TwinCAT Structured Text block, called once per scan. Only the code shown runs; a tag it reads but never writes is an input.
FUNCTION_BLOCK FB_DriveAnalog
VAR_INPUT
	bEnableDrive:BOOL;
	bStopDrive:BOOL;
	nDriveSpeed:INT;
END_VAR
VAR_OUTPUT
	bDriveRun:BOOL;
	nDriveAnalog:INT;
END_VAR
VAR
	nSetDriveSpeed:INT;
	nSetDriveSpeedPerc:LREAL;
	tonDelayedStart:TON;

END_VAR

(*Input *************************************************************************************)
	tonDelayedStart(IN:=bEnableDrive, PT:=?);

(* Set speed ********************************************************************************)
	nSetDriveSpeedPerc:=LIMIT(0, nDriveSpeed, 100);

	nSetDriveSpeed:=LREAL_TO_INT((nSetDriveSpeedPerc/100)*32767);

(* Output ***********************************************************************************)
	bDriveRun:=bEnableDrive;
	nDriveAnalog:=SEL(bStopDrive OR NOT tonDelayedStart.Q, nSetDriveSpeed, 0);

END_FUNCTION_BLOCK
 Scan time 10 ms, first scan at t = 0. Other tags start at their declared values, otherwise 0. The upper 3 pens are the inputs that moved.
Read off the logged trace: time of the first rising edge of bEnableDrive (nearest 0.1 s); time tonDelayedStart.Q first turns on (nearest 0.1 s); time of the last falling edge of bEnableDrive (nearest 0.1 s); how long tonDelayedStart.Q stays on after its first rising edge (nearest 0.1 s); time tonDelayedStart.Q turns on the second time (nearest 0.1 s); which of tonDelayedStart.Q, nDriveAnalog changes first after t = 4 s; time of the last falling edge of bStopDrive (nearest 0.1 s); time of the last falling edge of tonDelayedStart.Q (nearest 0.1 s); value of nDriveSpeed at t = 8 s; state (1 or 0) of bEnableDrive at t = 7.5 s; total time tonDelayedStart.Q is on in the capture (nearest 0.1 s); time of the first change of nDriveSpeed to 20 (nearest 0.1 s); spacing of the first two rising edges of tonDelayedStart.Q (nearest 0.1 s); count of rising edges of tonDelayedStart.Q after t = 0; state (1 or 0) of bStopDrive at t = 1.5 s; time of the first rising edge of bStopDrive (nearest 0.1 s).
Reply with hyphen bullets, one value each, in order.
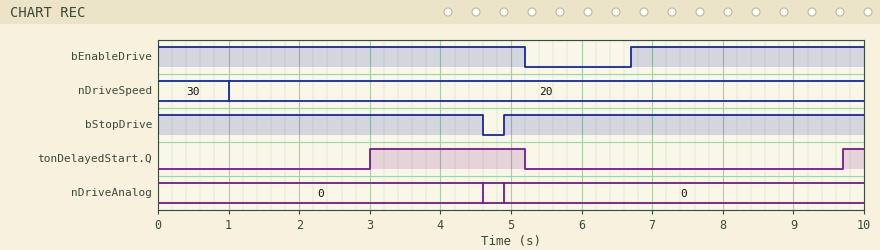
- 6.7 s
- 3.0 s
- 5.2 s
- 2.2 s
- 9.7 s
- nDriveAnalog
- 4.6 s
- 5.2 s
- 20
- 1
- 2.5 s
- 1.0 s
- 6.7 s
- 2
- 1
- 4.9 s
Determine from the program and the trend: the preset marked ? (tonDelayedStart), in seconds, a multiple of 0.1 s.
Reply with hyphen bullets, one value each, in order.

- 3.0 s
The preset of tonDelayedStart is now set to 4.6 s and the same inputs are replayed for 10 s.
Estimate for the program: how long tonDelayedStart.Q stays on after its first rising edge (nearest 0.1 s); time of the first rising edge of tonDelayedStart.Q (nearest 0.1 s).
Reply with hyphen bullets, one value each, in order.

- 0.6 s
- 4.6 s
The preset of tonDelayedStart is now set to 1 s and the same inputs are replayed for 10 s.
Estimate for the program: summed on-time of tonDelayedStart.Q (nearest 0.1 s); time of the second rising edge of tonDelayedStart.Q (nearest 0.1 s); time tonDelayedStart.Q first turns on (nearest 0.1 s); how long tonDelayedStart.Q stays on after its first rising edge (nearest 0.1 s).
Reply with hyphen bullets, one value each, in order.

- 6.5 s
- 7.7 s
- 1.0 s
- 4.2 s
